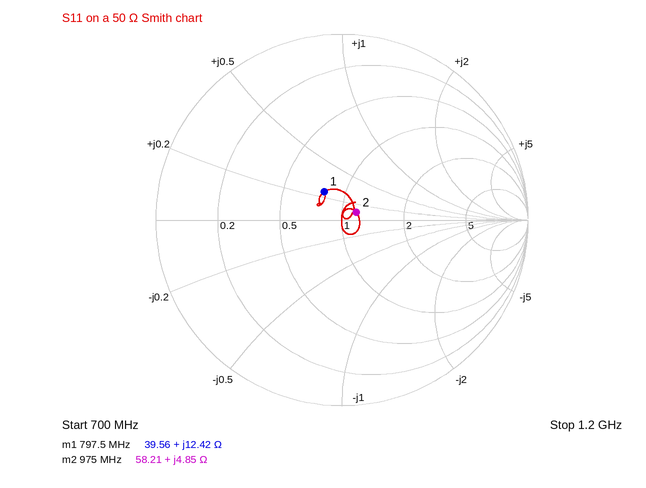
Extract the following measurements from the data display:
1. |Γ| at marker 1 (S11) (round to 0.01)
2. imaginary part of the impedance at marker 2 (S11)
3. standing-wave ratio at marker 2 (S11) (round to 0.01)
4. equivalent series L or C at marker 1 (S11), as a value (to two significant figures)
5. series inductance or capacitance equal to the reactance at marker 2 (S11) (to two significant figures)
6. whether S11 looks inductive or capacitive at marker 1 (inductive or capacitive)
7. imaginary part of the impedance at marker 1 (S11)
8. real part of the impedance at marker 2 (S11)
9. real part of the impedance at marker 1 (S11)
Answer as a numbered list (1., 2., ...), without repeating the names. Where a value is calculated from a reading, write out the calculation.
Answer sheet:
1. 0.18
2. +4.85 Ω
3. 1.19
4. L = 12.42 Ω/(2π × 797.5 MHz) ≈ 2.5 nH
5. L = 4.85 Ω/(2π × 975 MHz) ≈ 792 pH, so 790 pH to two significant figures
6. inductive
7. +12.42 Ω
8. 58.21 Ω
9. 39.56 Ω
